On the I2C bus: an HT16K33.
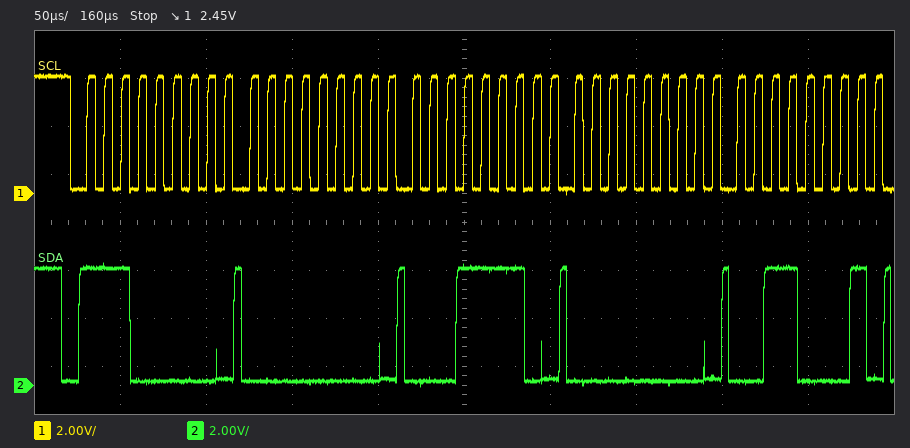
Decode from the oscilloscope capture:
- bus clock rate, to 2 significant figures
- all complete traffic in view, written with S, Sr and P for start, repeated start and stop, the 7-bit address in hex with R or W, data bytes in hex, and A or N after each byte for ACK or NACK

100 kHz
S 70W A 00 A 1E A 00 A 31 A
